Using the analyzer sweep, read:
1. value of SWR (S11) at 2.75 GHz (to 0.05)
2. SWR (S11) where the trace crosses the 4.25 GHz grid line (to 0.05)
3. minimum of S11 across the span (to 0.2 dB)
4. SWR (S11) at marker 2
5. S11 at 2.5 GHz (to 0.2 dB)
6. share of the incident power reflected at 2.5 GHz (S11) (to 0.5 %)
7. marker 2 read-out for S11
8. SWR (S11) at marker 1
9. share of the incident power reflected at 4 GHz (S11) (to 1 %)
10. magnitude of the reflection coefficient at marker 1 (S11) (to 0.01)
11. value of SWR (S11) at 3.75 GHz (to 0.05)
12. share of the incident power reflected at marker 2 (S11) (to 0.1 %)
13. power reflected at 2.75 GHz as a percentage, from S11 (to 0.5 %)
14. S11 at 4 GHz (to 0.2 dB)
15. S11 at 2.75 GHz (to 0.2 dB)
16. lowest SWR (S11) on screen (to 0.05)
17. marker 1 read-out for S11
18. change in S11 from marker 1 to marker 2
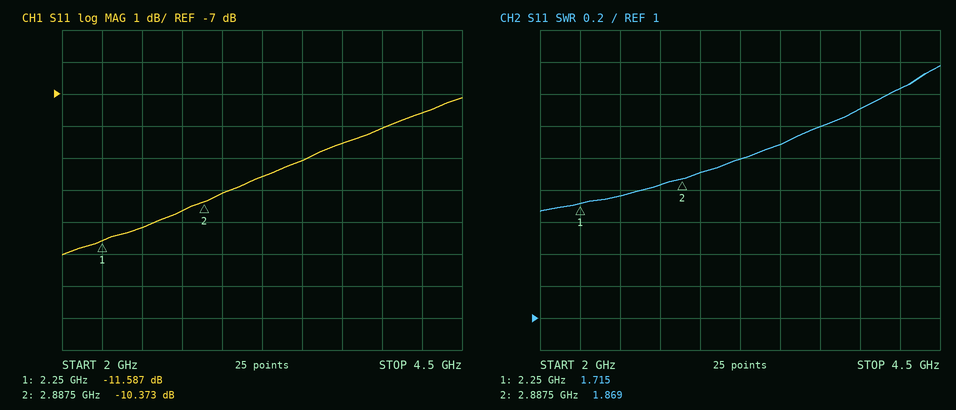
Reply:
1.85
2.45
-12.0 dB
1.869
-11.2 dB
7.5 %
-10.373 dB
1.715
16 %
0.26
2.20
9.2 %
8.5 %
-8.0 dB
-10.6 dB
1.65
-11.587 dB
1.214 dB
